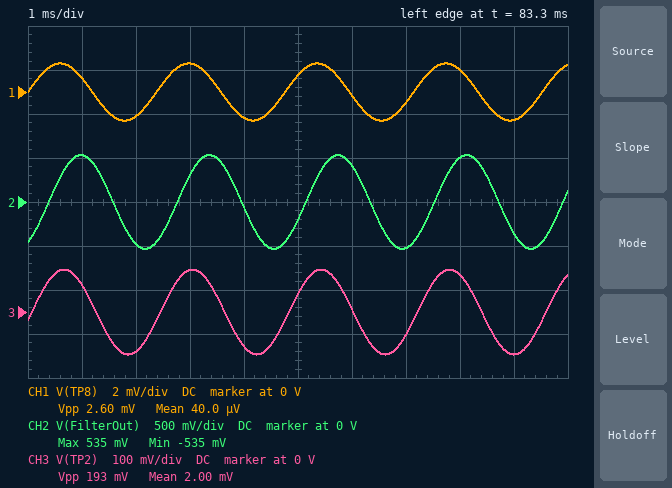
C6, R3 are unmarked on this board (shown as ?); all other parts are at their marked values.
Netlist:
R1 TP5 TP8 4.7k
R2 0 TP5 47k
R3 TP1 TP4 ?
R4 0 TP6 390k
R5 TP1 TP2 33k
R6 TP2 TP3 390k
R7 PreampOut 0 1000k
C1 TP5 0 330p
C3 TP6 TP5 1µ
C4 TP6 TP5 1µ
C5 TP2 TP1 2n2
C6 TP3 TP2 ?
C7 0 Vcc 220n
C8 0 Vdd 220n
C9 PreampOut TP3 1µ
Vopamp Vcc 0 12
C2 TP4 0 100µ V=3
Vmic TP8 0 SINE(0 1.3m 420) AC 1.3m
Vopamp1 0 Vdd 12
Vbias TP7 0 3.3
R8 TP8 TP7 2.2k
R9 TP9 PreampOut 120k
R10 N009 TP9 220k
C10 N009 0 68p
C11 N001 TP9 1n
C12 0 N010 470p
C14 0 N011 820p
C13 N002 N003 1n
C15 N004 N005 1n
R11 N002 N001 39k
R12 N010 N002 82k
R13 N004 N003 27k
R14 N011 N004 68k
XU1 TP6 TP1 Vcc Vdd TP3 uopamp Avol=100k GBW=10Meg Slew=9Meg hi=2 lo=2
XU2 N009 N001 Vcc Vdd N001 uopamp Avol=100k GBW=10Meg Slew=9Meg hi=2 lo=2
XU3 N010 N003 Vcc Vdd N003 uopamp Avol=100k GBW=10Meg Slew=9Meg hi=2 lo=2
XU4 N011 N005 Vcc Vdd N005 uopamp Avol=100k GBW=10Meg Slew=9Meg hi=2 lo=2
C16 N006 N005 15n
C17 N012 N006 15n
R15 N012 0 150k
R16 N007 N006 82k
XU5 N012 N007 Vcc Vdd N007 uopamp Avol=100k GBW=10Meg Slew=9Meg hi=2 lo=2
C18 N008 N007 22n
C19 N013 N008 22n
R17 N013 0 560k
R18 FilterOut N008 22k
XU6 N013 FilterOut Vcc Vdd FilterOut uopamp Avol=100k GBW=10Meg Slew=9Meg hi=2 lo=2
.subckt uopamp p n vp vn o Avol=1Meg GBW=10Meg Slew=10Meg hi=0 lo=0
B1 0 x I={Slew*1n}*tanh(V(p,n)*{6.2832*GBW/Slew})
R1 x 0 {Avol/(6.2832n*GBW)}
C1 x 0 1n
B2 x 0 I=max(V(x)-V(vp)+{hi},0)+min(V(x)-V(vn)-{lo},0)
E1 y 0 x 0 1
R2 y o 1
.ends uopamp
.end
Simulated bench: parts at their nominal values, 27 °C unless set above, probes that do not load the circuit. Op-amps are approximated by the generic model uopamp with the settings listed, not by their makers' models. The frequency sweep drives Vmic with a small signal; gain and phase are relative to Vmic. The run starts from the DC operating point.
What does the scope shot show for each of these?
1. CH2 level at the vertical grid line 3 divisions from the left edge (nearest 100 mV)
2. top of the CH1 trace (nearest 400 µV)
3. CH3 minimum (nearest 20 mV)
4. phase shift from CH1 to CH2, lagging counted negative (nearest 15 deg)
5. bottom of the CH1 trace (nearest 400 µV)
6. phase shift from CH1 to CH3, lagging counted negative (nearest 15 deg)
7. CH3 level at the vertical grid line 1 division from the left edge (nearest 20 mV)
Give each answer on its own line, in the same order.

300 mV
1.2 mV
-100 mV
-60 deg
-1.2 mV
-15 deg
60 mV
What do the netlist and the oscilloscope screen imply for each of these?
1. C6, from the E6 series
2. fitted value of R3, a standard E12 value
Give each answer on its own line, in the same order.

2.2 nF
390 Ω
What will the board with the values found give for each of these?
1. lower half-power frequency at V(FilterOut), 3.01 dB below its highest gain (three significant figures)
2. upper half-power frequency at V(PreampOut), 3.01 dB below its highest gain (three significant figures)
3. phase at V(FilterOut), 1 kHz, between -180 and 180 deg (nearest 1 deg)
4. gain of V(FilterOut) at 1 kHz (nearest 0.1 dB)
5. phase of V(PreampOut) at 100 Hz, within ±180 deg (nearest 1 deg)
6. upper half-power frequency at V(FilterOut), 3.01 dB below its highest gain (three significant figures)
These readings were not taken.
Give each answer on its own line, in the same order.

61.1 Hz
195 Hz
-112 deg
46.3 dB
-24 deg
175 Hz
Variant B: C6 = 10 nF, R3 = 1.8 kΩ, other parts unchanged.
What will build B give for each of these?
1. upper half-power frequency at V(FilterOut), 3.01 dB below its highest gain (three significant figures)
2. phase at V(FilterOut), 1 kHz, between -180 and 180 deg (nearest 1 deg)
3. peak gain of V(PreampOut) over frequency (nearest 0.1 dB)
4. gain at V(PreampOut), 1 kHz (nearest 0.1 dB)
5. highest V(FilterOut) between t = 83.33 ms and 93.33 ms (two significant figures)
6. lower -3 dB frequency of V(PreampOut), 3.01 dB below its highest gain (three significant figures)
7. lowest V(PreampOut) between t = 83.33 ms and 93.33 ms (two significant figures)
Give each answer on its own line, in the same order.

104 Hz
-92 deg
46.3 dB
26.2 dB
38 mV
913 mHz
-38 mV
